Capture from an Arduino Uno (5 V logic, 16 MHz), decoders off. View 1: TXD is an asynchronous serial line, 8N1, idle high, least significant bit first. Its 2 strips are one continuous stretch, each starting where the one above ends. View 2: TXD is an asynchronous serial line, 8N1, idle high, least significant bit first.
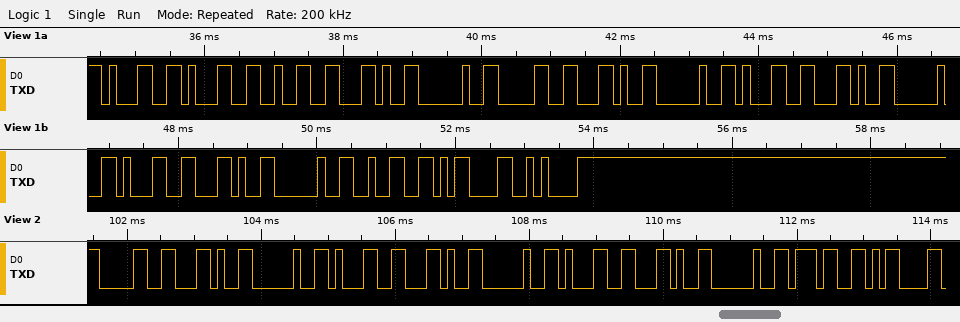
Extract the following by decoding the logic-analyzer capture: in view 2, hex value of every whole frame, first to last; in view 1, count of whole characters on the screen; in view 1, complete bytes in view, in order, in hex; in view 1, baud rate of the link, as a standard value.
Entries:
30 2C 20 31 2C 20 31 2C 20 37 0D
17
31 31 32 2C 20 30 2C 20 31 2C 20 31 2C 20 32 0D 0A
9600 baud
